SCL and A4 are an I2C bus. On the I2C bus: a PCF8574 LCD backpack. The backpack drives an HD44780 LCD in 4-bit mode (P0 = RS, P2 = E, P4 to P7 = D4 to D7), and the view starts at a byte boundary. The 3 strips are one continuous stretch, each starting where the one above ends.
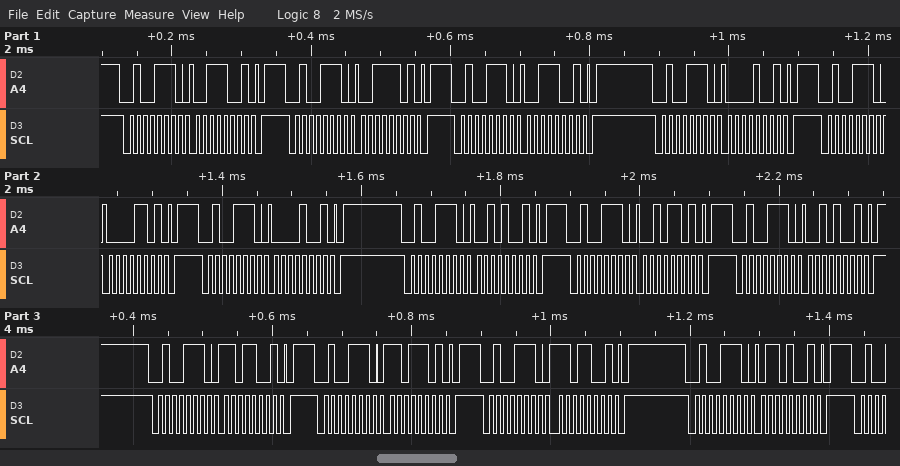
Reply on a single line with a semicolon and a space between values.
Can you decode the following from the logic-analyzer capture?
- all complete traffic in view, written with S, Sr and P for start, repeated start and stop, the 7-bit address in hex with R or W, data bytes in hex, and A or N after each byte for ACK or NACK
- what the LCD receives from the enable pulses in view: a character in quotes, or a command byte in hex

S 27W A 39 A P S 27W A 3D A P S 27W A 39 A P S 27W A 09 A P S 27W A 0D A P S 27W A 09 A P S 27W A 29 A P S 27W A 2D A P S 27W A 29 A P S 27W A D9 A P S 27W A DD A P S 27W A D9 A P S 27W A 69 A P; '0' '-'
